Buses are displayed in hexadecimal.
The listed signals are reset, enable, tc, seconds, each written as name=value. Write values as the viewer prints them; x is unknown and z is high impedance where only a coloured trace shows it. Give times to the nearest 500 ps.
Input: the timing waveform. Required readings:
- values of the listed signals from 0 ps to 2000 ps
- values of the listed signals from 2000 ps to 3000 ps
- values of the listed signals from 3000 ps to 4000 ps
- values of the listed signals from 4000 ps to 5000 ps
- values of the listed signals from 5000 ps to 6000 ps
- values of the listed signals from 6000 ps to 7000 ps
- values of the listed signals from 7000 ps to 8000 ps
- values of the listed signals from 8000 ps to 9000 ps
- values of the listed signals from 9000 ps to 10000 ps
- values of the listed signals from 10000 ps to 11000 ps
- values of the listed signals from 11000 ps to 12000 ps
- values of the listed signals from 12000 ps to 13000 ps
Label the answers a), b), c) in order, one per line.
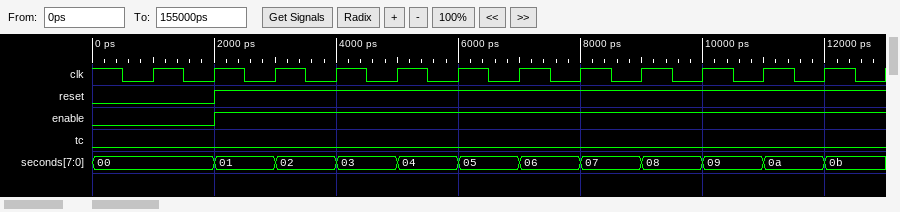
a) reset=0, enable=0, tc=0, seconds=00
b) reset=1, enable=1, tc=0, seconds=01
c) reset=1, enable=1, tc=0, seconds=02
d) reset=1, enable=1, tc=0, seconds=03
e) reset=1, enable=1, tc=0, seconds=04
f) reset=1, enable=1, tc=0, seconds=05
g) reset=1, enable=1, tc=0, seconds=06
h) reset=1, enable=1, tc=0, seconds=07
i) reset=1, enable=1, tc=0, seconds=08
j) reset=1, enable=1, tc=0, seconds=09
k) reset=1, enable=1, tc=0, seconds=0a
l) reset=1, enable=1, tc=0, seconds=0b
